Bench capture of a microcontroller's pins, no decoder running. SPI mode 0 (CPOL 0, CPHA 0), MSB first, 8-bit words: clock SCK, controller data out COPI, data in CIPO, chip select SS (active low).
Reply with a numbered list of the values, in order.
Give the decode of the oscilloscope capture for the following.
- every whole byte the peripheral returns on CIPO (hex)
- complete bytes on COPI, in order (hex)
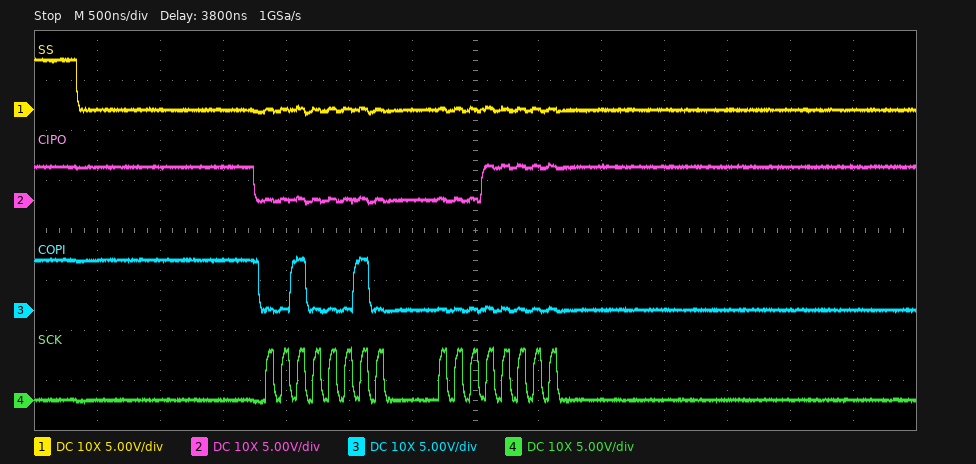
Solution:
1. 00 1F
2. 22 00
